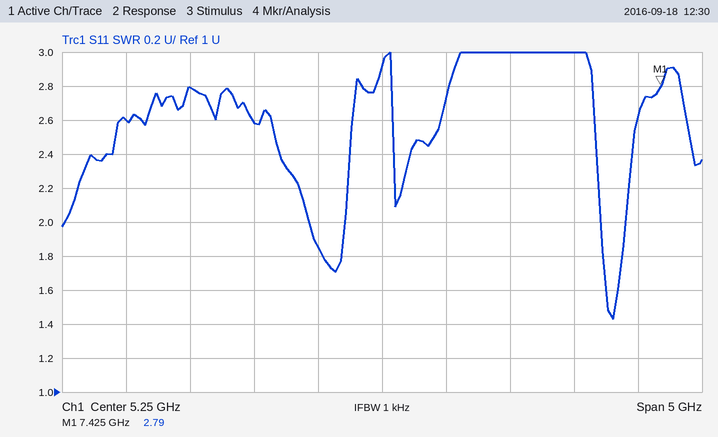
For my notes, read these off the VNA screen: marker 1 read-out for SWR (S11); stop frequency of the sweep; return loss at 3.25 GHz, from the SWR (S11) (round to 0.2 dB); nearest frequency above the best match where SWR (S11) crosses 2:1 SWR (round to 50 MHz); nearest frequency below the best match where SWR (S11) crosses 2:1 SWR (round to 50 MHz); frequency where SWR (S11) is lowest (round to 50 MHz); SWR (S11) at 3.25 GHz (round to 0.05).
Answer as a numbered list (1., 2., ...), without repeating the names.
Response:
1. 2.79
2. 7.75 GHz
3. 7.0 dB
4. 7.15 GHz
5. 6.95 GHz
6. 7.05 GHz
7. 2.60
